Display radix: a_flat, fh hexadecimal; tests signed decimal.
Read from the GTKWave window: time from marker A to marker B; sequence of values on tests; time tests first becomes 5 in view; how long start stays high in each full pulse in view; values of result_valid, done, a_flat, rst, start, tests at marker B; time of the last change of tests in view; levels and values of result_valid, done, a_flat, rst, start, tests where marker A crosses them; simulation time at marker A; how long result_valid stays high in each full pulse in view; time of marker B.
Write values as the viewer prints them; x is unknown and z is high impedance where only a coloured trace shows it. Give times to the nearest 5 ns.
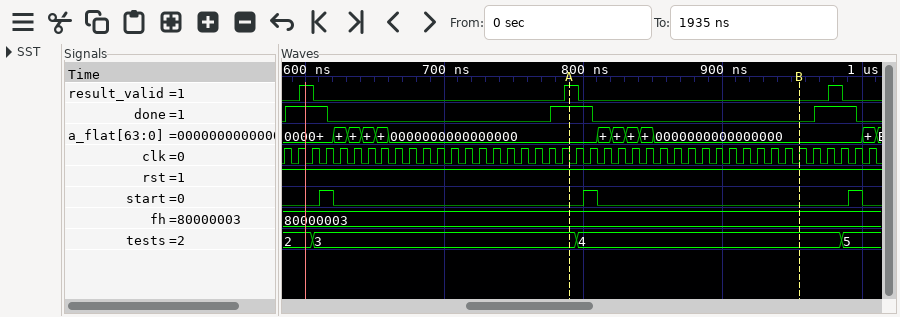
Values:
165 ns
2, 3, 4, 5
985 ns
10 ns, 10 ns, 10 ns
result_valid=0, done=0, a_flat=0000000000000000, rst=1, start=0, tests=4
985 ns
result_valid=1, done=1, a_flat=0000000000000000, rst=1, start=0, tests=3
790 ns
10 ns, 10 ns, 10 ns
955 ns
